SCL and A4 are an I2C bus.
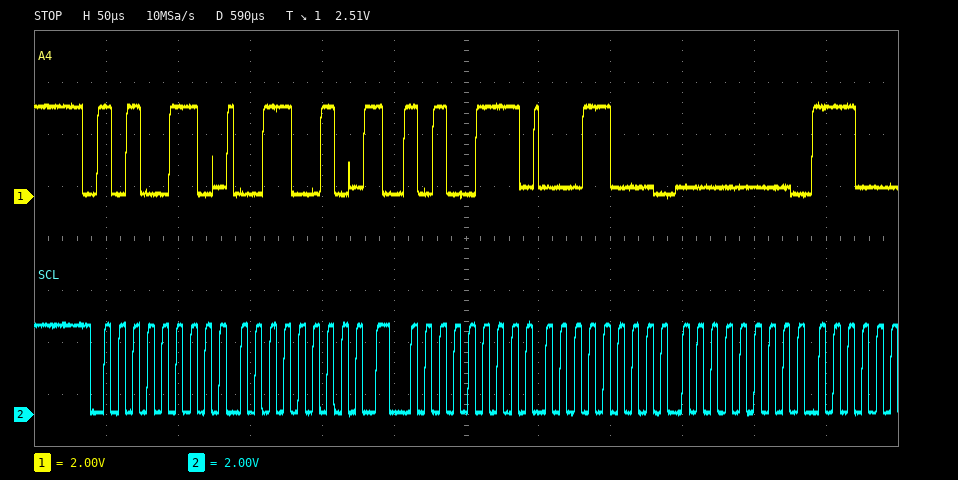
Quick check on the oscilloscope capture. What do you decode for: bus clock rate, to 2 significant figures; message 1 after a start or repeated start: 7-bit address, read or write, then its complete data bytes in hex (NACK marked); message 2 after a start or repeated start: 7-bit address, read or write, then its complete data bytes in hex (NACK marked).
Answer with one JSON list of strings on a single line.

["100 kHz", "0x53 write: 32", "0x53 read: 18 00"]
